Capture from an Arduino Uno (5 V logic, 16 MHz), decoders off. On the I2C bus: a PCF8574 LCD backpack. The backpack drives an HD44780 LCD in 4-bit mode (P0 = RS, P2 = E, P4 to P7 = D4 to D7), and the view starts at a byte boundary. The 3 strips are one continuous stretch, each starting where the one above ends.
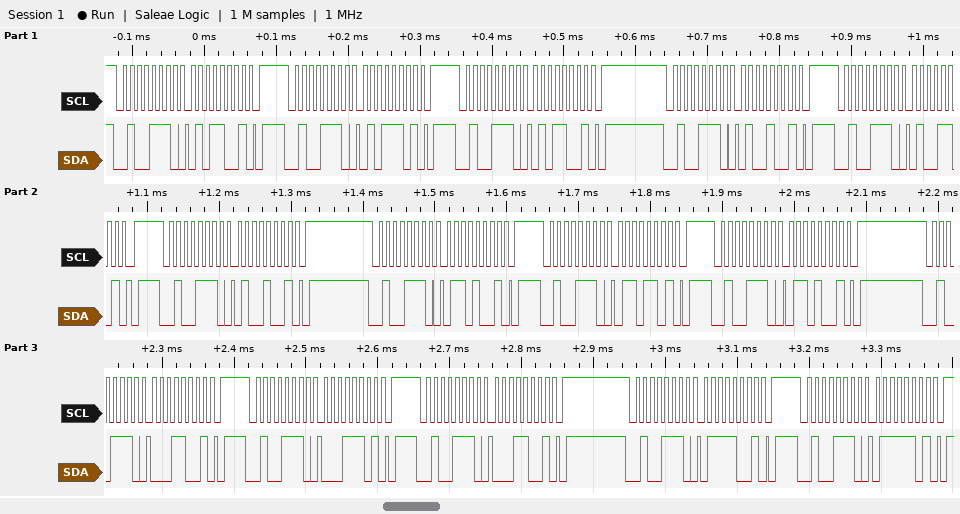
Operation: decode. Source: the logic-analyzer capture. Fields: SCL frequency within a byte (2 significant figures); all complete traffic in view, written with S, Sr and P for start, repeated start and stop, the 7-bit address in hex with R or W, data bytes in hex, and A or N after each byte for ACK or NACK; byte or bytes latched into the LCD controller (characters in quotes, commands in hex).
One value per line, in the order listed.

100 kHz
S 27W A 59 A P S 27W A 5D A P S 27W A 59 A P S 27W A 49 A P S 27W A 4D A P S 27W A 49 A P S 27W A 69 A P S 27W A 6D A P S 27W A 69 A P S 27W A 19 A P S 27W A 1D A P S 27W A 19 A P S 27W A 79 A P S 27W A 7D A P
'T' 'a'
